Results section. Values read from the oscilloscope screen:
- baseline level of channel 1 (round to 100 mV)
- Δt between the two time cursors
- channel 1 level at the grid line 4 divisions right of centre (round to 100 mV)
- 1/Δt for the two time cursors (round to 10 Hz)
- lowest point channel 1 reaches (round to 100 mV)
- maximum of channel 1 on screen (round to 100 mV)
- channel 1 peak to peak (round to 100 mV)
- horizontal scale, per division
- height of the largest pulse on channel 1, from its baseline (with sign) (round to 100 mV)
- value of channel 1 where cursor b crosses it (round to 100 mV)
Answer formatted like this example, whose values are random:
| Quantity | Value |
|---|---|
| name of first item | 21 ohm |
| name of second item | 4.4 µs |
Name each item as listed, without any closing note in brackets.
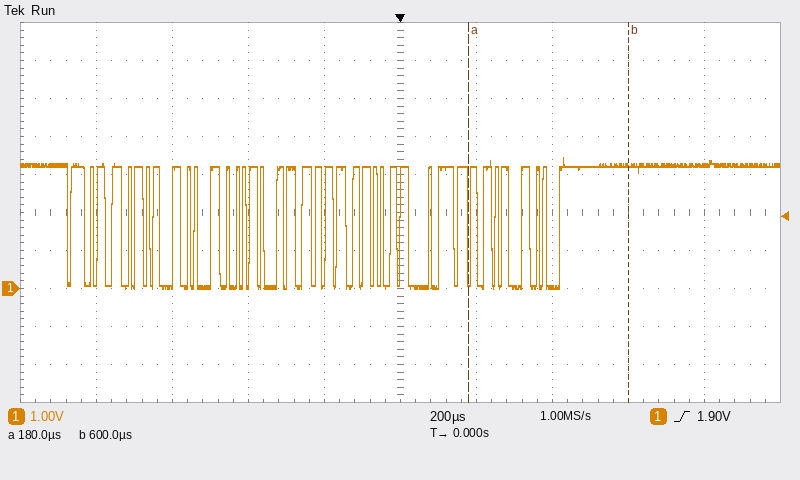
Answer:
| Quantity | Value |
|---|---|
| baseline level of channel 1 | 3.2 V |
| Δt between the two time cursors | 420 µs |
| channel 1 level at the grid line 4 divisions right of centre | 3.2 V |
| 1/Δt for the two time cursors | 2.38 kHz |
| lowest point channel 1 reaches | 0.0 V |
| maximum of channel 1 on screen | 3.4 V |
| channel 1 peak to peak | 3.4 V |
| horizontal scale, per division | 200 µs |
| height of the largest pulse on channel 1, from its baseline (with sign) | -3.2 V |
| value of channel 1 where cursor b crosses it | 3.2 V |
